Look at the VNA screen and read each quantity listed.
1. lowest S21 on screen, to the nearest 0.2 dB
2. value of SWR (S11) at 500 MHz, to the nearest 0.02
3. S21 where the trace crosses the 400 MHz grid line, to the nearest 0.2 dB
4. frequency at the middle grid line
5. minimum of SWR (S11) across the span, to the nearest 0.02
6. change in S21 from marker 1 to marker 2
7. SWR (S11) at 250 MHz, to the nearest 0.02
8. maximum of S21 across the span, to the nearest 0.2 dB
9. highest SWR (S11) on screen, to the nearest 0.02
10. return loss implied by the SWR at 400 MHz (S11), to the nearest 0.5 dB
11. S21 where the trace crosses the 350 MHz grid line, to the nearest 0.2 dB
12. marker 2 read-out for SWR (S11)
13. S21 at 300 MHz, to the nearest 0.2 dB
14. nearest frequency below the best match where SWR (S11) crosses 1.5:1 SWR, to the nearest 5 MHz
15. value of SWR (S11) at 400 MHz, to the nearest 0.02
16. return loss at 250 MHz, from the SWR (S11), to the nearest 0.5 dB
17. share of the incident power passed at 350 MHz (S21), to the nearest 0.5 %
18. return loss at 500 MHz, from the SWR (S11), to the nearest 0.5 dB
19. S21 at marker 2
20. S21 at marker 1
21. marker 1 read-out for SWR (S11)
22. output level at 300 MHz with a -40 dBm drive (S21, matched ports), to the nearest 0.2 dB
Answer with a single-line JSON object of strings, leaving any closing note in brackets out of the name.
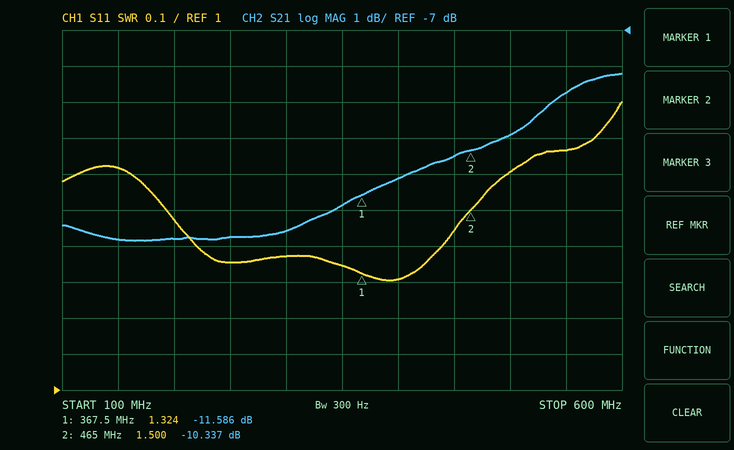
{"lowest S21 on screen, to the nearest 0.2 dB": "-12.8 dB", "value of SWR (S11) at 500 MHz, to the nearest 0.02": "1.60", "S21 where the trace crosses the 400 MHz grid line, to the nearest 0.2 dB": "-11.2 dB", "frequency at the middle grid line": "350 MHz", "minimum of SWR (S11) across the span, to the nearest 0.02": "1.30", "change in S21 from marker 1 to marker 2": "1.249 dB", "SWR (S11) at 250 MHz, to the nearest 0.02": "1.36", "maximum of S21 across the span, to the nearest 0.2 dB": "-8.2 dB", "highest SWR (S11) on screen, to the nearest 0.02": "1.80", "return loss implied by the SWR at 400 MHz (S11), to the nearest 0.5 dB": "17.5 dB", "S21 where the trace crosses the 350 MHz grid line, to the nearest 0.2 dB": "-11.8 dB", "marker 2 read-out for SWR": "1.500", "S21 at 300 MHz, to the nearest 0.2 dB": "-12.6 dB", "nearest frequency below the best match where SWR (S11) crosses 1.5:1 SWR, to the nearest 5 MHz": "195 MHz", "value of SWR (S11) at 400 MHz, to the nearest 0.02": "1.30", "return loss at 250 MHz, from the SWR (S11), to the nearest 0.5 dB": "16.5 dB", "share of the incident power passed at 350 MHz (S21), to the nearest 0.5 %": "6.5 %", "return loss at 500 MHz, from the SWR (S11), to the nearest 0.5 dB": "12.5 dB", "S21 at marker 2": "-10.337 dB", "S21 at marker 1": "-11.586 dB", "marker 1 read-out for SWR": "1.324", "output level at 300 MHz with a -40 dBm drive (S21, matched ports), to the nearest 0.2 dB": "-52.6 dBm"}
